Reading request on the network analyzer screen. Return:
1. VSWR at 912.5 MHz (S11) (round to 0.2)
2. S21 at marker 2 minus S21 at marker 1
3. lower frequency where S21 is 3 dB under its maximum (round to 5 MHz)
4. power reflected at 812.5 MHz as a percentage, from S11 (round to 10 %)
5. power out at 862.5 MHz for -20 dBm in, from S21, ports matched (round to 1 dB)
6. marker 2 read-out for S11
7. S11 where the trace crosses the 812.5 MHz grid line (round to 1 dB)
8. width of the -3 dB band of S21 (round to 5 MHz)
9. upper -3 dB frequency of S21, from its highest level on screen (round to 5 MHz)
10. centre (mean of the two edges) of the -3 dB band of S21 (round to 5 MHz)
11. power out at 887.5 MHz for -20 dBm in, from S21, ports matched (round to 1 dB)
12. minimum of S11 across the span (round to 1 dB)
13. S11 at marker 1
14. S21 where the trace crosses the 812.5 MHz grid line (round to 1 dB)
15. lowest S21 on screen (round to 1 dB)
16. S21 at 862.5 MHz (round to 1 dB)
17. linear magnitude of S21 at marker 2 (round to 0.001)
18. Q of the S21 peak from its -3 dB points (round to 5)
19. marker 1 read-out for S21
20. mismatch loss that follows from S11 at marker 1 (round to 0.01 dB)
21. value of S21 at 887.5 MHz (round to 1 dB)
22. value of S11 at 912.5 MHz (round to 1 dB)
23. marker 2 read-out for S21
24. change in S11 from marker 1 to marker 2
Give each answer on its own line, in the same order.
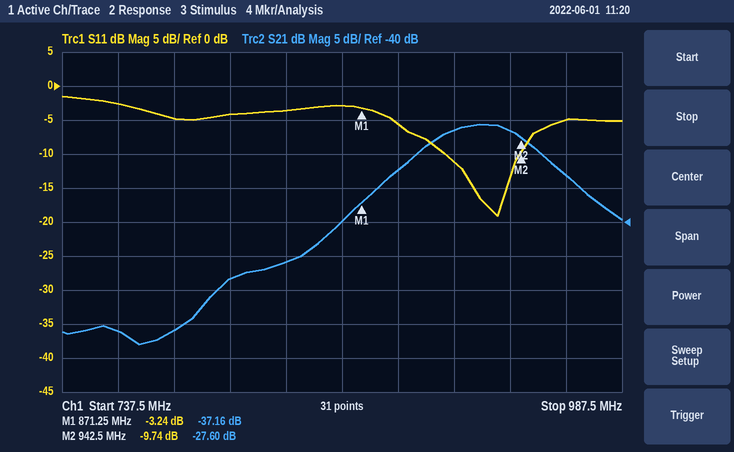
1.8
9.56 dB
900 MHz
40 %
-60 dBm
-9.74 dB
-4 dB
45 MHz
945 MHz
925 MHz
-52 dBm
-19 dB
-3.24 dB
-48 dB
-58 dB
-40 dB
0.042
20
-37.16 dB
2.79 dB
-32 dB
-11 dB
-27.60 dB
-6.50 dB
